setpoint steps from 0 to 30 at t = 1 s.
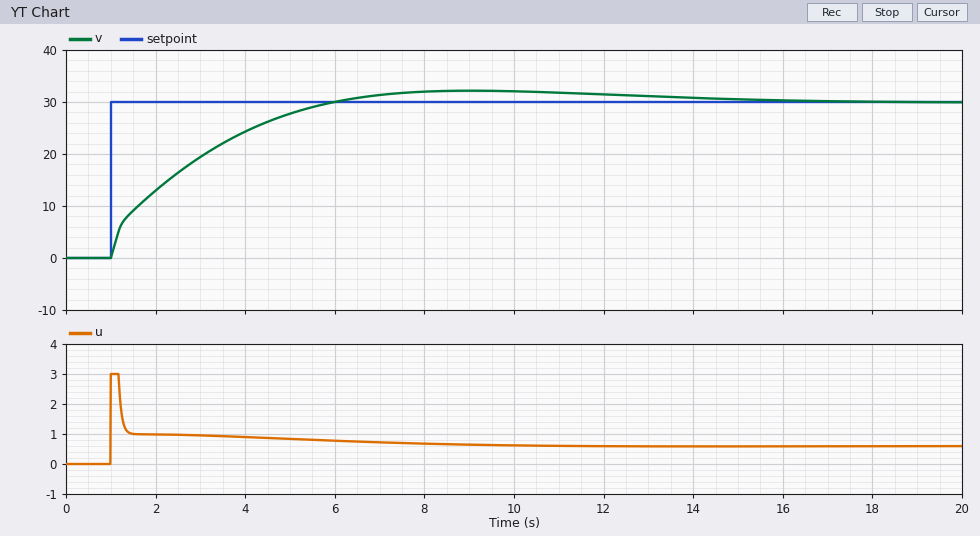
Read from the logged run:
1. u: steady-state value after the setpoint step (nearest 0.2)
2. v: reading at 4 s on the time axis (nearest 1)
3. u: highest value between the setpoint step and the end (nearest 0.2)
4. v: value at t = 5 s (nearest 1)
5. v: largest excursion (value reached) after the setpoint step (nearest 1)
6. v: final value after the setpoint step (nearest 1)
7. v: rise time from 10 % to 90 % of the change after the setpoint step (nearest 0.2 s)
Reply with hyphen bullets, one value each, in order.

- 0.6
- 24
- 3.0
- 28
- 32
- 30
- 3.6 s
